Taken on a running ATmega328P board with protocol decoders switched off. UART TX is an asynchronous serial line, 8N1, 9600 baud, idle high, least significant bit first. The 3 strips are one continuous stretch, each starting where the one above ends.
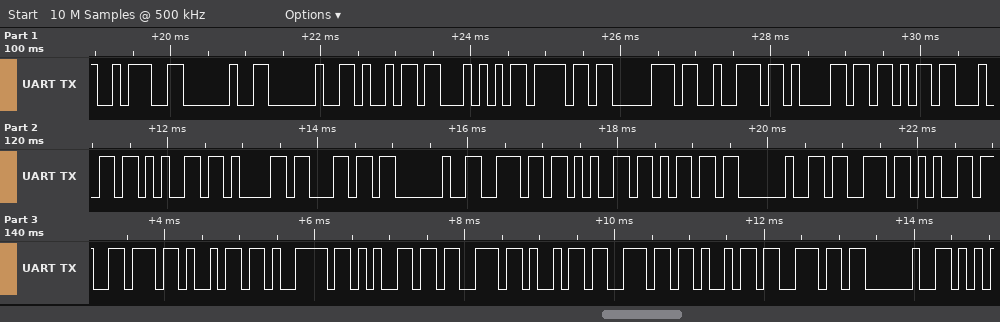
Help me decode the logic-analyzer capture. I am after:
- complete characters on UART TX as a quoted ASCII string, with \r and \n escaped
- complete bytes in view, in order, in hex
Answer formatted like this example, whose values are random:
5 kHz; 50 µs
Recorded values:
":  iToprakdeal nem seviyesinin "; 3A 20 20 69 54 6F 70 72 61 6B 64 65 61 6C 20 6E 65 6D 20 73 65 76 69 79 65 73 69 6E 69 6E 20
